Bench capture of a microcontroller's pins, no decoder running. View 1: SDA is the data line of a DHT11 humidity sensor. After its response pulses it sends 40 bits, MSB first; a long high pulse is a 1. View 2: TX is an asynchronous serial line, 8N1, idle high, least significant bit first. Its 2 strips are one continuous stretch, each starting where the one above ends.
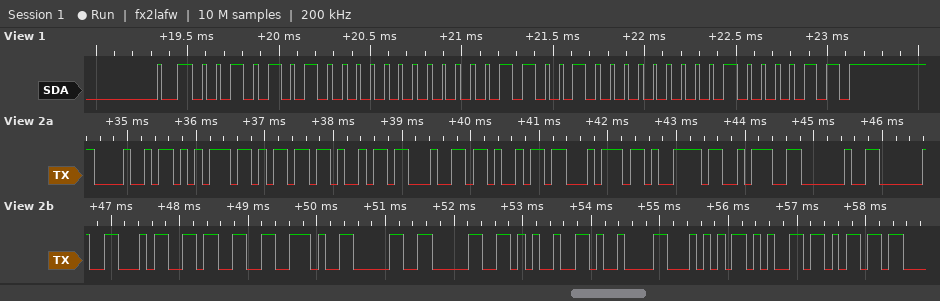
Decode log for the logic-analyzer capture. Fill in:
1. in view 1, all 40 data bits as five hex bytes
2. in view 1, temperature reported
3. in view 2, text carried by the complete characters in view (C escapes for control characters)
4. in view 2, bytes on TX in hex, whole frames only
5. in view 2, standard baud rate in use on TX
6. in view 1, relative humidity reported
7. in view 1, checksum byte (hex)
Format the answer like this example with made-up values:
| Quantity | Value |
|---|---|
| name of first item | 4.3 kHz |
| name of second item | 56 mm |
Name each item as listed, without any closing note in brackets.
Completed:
| Quantity | Value |
|---|---|
| in view 1, all 40 data bits as five hex bytes | 2A 00 19 00 43 |
| in view 1, temperature reported | 25.0 °C |
| in view 2, text carried by the complete characters in view | "Humidity:  43.00%\tTem" |
| in view 2, bytes on TX in hex, whole frames only | 0x48 0x75 0x6D 0x69 0x64 0x69 0x74 0x79 0x3A 0x20 0x20 0x34 0x33 0x2E 0x30 0x30 0x25 0x09 0x54 0x65 0x6D |
| in view 2, standard baud rate in use on TX | 9600 baud |
| in view 1, relative humidity reported | 42 % |
| in view 1, checksum byte | 0x43 |
